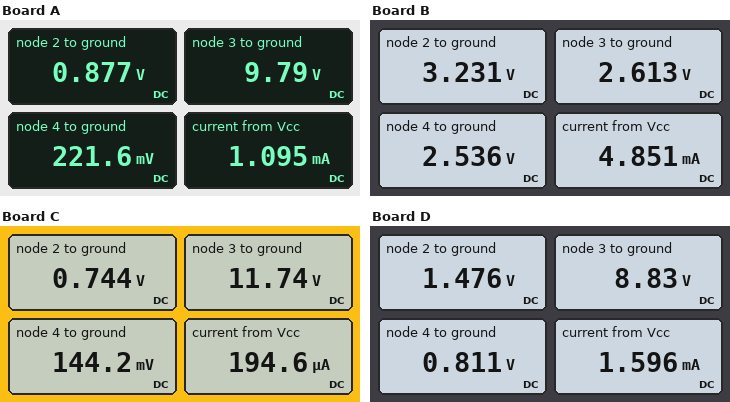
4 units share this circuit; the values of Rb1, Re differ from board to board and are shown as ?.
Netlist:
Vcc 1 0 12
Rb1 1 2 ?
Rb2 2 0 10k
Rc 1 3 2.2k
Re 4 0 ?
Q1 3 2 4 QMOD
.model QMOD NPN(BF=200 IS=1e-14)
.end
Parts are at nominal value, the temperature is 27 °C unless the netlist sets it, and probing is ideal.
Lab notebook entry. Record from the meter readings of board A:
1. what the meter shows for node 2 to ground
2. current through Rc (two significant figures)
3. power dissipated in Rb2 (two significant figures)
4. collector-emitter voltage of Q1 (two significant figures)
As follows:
0.877 V
1.0 mA
77 µW
9.6 V
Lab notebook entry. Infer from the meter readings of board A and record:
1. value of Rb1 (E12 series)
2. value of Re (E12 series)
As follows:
120 kΩ
220 Ω
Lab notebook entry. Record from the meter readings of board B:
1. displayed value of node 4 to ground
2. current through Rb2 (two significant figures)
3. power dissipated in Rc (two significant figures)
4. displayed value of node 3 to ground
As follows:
2.536 V
320 µA
40 mW
2.613 V
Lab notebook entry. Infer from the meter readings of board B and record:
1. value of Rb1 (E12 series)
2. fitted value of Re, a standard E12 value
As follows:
15 kΩ
560 Ω
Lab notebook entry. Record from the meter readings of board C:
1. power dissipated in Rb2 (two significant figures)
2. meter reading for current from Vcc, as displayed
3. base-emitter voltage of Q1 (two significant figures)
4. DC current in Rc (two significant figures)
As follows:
55 µW
194.6 µA
600 mV
120 µA
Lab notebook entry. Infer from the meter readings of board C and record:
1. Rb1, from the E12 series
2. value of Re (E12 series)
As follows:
150 kΩ
1.2 kΩ
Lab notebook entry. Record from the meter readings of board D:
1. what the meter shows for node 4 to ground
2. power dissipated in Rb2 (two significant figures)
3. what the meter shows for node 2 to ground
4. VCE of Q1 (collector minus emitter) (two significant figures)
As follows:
0.811 V
220 µW
1.476 V
8.0 V
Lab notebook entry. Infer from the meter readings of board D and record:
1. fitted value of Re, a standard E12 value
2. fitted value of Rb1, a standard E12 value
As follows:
560 Ω
68 kΩ
